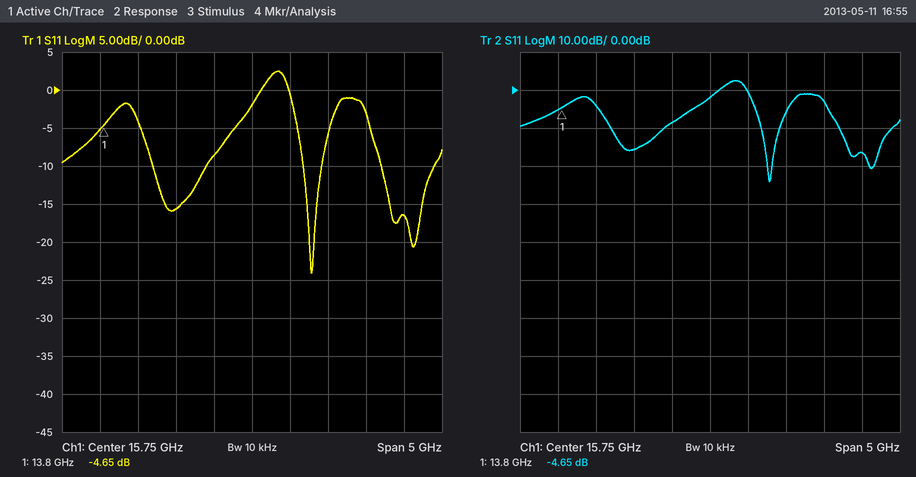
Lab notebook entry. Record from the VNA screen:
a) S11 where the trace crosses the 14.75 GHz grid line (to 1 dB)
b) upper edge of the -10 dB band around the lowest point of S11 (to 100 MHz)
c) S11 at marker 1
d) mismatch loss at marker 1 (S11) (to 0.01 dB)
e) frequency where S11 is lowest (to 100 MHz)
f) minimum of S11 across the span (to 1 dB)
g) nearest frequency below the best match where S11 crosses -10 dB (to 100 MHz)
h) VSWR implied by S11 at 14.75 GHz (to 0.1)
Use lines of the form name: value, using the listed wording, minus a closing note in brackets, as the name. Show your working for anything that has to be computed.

S11 where the trace crosses the 14.75 GHz grid line: -16 dB
upper edge of the -10 dB band around the lowest point of S11: 16.7 GHz
S11 at marker 1: -4.65 dB
mismatch loss at marker 1 (S11): −10 log10(1 − 10^(-4.65/10)) ≈ 1.82 dB
frequency where S11 is lowest: 16.5 GHz
minimum of S11 across the span: -24 dB
nearest frequency below the best match where S11 crosses -10 dB: 16.4 GHz
VSWR implied by S11 at 14.75 GHz: |Γ| = 10^(-16/20) = 0.1585; VSWR = (1 + 0.1585)/(1 − 0.1585) ≈ 1.4
